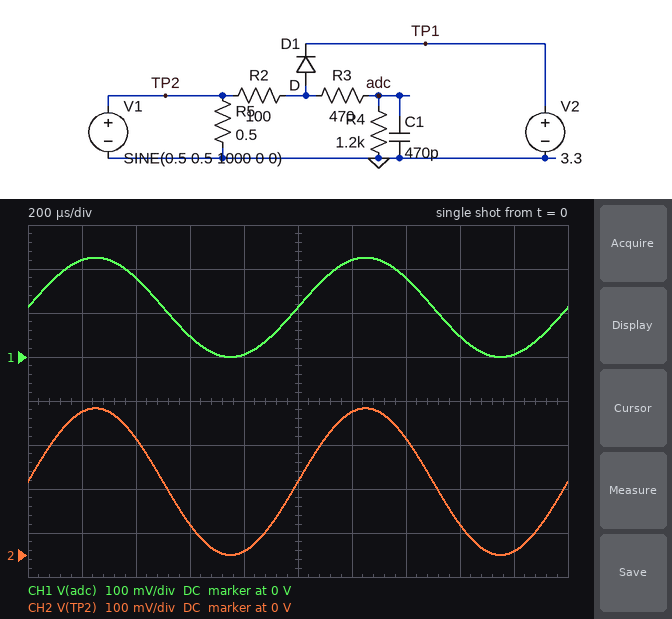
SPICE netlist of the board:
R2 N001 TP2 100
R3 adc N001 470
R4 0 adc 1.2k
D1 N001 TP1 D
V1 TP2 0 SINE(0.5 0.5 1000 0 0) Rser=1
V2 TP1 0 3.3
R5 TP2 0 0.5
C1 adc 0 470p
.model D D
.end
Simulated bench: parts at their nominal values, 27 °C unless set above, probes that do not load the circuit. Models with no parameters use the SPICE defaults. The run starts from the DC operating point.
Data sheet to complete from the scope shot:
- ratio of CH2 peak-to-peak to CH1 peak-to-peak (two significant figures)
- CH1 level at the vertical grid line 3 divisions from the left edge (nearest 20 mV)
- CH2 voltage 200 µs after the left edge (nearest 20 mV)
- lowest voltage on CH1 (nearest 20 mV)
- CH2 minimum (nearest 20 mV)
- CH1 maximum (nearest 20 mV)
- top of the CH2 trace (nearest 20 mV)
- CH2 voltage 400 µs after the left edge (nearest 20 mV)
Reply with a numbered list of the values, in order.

1. 1.5
2. 40 mV
3. 320 mV
4. 0 V
5. 0 V
6. 220 mV
7. 340 mV
8. 260 mV
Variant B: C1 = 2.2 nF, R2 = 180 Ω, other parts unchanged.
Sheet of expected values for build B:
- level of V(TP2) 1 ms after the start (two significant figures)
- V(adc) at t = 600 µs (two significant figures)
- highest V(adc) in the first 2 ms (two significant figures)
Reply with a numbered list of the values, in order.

1. 170 mV
2. 45 mV
3. 220 mV
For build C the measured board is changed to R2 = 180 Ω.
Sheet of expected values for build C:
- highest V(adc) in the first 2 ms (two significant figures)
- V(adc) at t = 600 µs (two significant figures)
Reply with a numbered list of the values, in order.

1. 220 mV
2. 45 mV
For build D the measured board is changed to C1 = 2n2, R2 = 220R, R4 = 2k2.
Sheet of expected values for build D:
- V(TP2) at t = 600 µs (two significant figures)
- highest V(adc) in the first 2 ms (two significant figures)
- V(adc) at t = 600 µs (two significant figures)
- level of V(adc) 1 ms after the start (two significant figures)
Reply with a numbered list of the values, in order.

1. 69 mV
2. 250 mV
3. 53 mV
4. 130 mV
